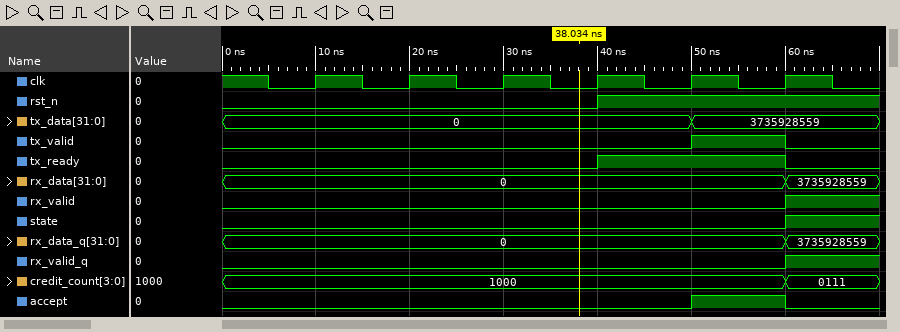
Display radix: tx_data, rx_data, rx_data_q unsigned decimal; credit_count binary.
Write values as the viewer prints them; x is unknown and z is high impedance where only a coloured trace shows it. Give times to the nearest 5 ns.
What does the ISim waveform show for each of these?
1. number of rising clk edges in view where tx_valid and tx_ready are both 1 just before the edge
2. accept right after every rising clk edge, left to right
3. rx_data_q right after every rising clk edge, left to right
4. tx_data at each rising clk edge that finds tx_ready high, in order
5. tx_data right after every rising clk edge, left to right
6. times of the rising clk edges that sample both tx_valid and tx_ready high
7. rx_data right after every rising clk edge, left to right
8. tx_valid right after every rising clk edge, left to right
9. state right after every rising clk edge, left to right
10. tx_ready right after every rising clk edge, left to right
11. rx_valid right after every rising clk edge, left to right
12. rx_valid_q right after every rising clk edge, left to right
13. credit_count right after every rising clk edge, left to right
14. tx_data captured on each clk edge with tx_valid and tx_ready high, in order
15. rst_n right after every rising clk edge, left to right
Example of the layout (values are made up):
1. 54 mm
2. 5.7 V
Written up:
1. 1
2. 0 0 0 0 1 0
3. 0, 0, 0, 0, 0, 3735928559
4. 0, 3735928559
5. 0, 0, 0, 0, 3735928559, 3735928559
6. 60 ns
7. 0, 0, 0, 0, 0, 3735928559
8. 0 0 0 0 1 0
9. 0 0 0 0 0 1
10. 0 0 0 1 1 0
11. 0 0 0 0 0 1
12. 0 0 0 0 0 1
13. 1000, 1000, 1000, 1000, 1000, 0111
14. 3735928559
15. 0 0 0 1 1 1
